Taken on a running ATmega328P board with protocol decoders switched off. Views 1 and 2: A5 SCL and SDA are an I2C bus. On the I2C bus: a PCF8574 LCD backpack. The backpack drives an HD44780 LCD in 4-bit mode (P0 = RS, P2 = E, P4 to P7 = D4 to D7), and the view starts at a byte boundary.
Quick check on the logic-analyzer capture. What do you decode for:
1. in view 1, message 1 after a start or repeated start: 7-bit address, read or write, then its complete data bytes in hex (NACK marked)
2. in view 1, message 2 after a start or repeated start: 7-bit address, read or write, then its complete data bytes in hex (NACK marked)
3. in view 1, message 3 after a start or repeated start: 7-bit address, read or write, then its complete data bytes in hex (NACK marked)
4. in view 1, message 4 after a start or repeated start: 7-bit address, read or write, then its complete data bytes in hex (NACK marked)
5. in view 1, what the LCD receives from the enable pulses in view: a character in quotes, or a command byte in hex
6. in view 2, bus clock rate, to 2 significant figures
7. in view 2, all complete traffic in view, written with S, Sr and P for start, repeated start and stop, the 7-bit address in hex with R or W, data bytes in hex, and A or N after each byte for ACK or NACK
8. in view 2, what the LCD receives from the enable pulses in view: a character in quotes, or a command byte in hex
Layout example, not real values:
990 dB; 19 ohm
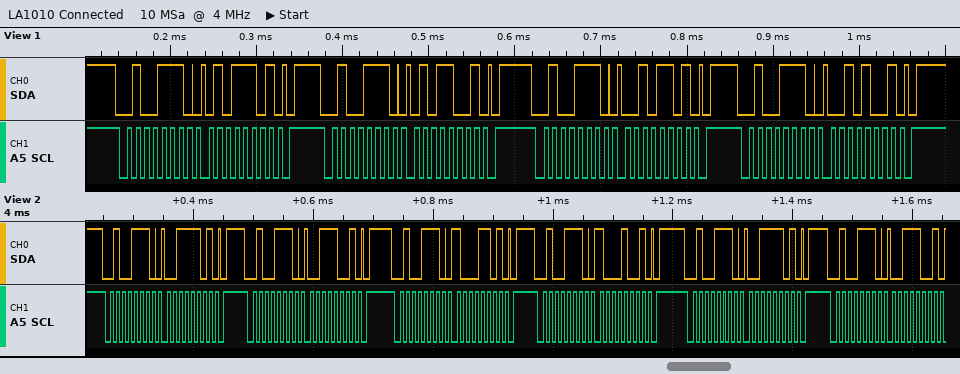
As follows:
0x27 write: 5D; 0x27 write: 59; 0x27 write: 2D; 0x27 write: 29; 'R'; 100 kHz; S 27W A 3D A P S 27W A 39 A P S 27W A 8D A P S 27W A 89 A P S 27W A 3D A P S 27W A 39 A; '8'
